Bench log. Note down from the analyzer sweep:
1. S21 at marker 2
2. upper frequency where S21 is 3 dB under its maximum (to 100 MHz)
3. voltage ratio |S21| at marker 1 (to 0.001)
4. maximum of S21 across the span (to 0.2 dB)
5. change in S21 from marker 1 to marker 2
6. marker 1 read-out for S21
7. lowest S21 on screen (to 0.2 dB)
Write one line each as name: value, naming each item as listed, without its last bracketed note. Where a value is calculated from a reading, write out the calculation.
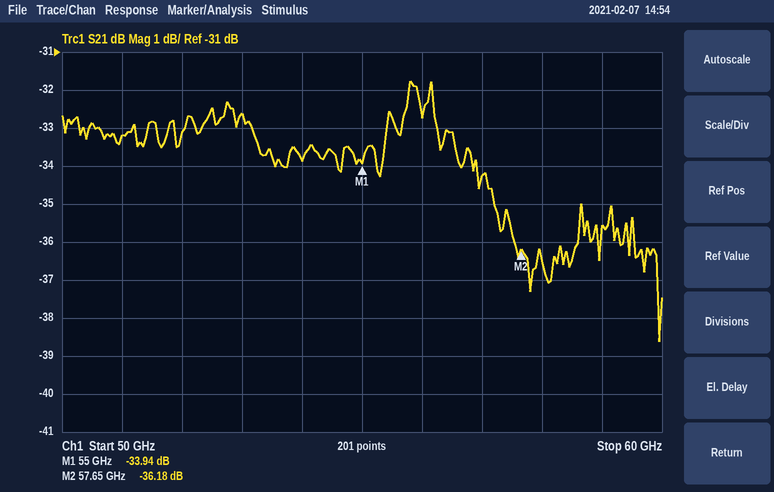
S21 at marker 2: -36.18 dB
upper frequency where S21 is 3 dB under its maximum: 57.2 GHz
voltage ratio |S21| at marker 1: 10^(-33.94/20) ≈ 0.020
maximum of S21 across the span: -31.8 dB
change in S21 from marker 1 to marker 2: -36.18 − (-33.94) = -2.24 dB
marker 1 read-out for S21: -33.94 dB
lowest S21 on screen: -38.6 dB
